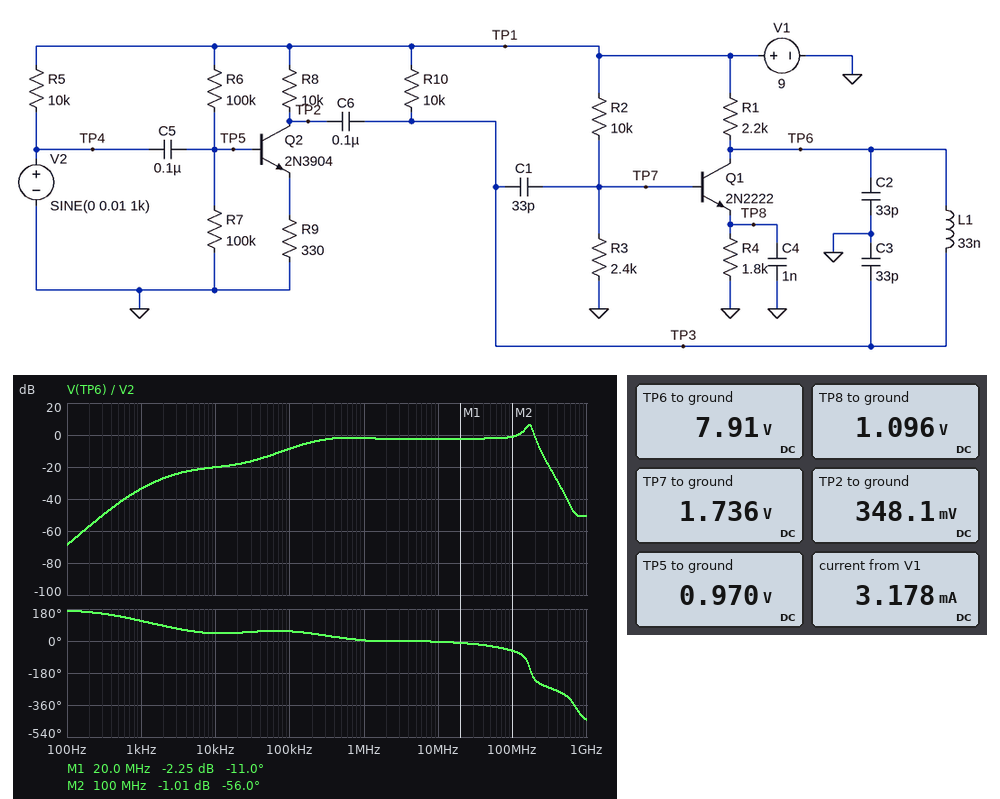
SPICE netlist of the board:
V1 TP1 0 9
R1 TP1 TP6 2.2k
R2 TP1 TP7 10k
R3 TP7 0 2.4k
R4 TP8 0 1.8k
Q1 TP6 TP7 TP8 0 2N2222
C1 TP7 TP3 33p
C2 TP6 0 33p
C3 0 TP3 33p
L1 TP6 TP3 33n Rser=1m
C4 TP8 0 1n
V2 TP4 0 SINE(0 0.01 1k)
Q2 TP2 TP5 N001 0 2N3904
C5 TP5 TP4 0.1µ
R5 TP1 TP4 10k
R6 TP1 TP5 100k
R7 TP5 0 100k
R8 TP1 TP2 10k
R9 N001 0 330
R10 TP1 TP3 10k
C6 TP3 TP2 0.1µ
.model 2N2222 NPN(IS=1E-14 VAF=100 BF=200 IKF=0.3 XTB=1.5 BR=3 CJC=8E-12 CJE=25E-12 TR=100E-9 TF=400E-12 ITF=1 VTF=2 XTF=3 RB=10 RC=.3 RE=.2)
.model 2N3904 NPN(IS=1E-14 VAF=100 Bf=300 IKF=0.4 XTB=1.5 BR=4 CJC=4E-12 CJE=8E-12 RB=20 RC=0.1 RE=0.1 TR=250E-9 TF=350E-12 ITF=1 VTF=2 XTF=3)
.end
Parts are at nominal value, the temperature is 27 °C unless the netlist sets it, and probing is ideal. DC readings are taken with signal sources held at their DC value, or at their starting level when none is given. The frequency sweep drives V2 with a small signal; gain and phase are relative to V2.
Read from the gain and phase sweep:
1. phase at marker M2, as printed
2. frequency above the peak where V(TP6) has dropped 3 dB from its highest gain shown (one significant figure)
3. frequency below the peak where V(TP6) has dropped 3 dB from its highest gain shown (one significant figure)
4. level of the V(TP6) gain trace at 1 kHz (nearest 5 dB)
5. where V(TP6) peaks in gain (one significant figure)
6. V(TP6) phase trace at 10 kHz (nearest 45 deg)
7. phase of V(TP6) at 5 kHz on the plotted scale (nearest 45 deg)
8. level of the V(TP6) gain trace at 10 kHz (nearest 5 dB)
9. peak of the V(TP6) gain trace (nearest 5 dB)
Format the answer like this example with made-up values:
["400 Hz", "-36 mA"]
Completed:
["-56.0 deg", "200 MHz", "100 MHz", "-35 dB", "200 MHz", "45 deg", "45 deg", "-20 dB", "5 dB"]
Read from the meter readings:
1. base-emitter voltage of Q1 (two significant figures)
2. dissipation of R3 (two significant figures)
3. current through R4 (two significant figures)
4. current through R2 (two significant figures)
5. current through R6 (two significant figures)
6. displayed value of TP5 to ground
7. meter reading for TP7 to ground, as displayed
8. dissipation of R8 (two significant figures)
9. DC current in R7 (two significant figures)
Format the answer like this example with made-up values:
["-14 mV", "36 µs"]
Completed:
["640 mV", "1.3 mW", "610 µA", "730 µA", "80 µA", "0.970 V", "1.736 V", "7.5 mW", "9.7 µA"]
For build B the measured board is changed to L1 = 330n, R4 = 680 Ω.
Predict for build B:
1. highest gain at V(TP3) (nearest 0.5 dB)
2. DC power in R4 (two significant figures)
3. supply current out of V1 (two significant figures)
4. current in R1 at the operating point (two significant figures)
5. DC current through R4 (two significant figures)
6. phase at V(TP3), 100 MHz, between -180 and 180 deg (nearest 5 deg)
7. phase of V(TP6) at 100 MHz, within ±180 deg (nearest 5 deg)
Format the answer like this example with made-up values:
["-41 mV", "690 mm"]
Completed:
["2.5 dB", "1.7 mW", "4.1 mA", "1.3 mA", "1.6 mA", "-30 deg", "75 deg"]
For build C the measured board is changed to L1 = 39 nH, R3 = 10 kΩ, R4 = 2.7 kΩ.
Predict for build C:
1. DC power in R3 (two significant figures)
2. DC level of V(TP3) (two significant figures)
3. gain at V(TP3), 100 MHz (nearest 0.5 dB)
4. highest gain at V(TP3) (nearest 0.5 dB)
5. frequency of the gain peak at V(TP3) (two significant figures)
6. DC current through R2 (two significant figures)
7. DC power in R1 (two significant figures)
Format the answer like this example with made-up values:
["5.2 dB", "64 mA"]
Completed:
["2.0 mW", "6.5 V", "-8.5 dB", "2.0 dB", "160 MHz", "450 µA", "2.9 mW"]
